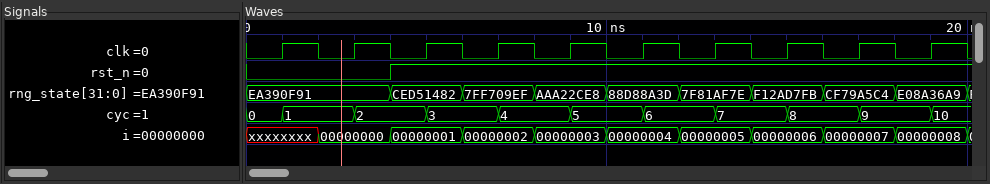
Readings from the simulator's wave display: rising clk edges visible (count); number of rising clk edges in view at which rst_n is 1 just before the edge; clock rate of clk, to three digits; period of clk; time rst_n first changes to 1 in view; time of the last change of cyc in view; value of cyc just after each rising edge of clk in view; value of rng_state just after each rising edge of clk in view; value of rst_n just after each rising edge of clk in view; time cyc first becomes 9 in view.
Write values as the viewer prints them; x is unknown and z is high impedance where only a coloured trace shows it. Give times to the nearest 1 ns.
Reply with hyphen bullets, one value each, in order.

- 10
- 8
- 500 MHz
- 2 ns
- 4 ns
- 19 ns
- 1, 2, 3, 4, 5, 6, 7, 8, 9, 10
- EA390F91, EA390F91, CED51482, 7FF709EF, AAA22CE8, 88D88A3D, 7F81AF7E, F12AD7FB, CF79A5C4, E08A36A9
- 0 0 1 1 1 1 1 1 1 1
- 17 ns
